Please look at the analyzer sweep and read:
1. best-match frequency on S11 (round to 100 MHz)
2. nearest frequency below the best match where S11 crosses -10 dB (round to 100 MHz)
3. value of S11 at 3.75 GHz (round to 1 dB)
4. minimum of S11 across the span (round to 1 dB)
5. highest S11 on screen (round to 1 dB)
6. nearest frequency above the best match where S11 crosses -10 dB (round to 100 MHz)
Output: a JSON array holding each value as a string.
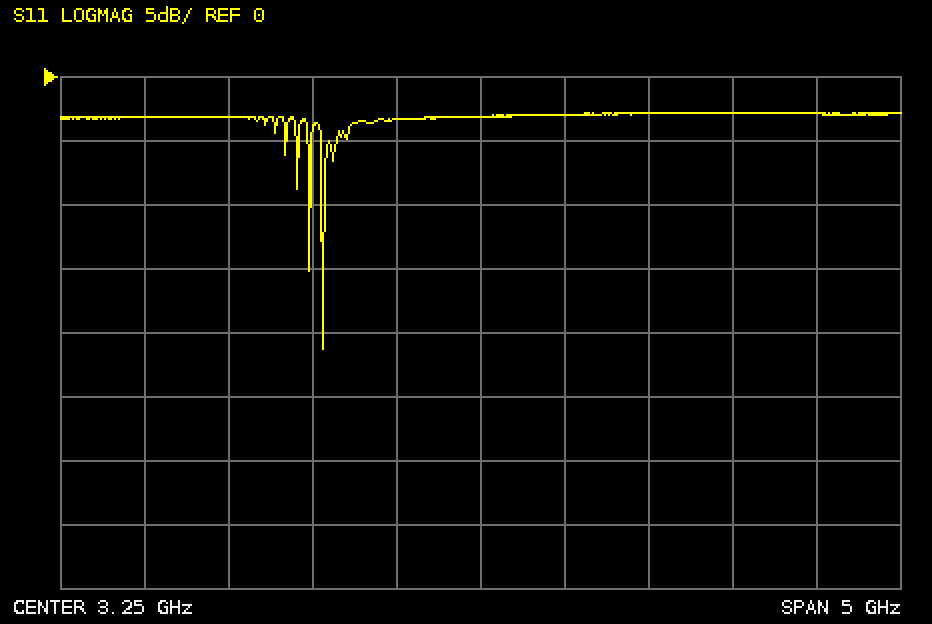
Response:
["2.3 GHz", "2.3 GHz", "-3 dB", "-21 dB", "-3 dB", "2.3 GHz"]
